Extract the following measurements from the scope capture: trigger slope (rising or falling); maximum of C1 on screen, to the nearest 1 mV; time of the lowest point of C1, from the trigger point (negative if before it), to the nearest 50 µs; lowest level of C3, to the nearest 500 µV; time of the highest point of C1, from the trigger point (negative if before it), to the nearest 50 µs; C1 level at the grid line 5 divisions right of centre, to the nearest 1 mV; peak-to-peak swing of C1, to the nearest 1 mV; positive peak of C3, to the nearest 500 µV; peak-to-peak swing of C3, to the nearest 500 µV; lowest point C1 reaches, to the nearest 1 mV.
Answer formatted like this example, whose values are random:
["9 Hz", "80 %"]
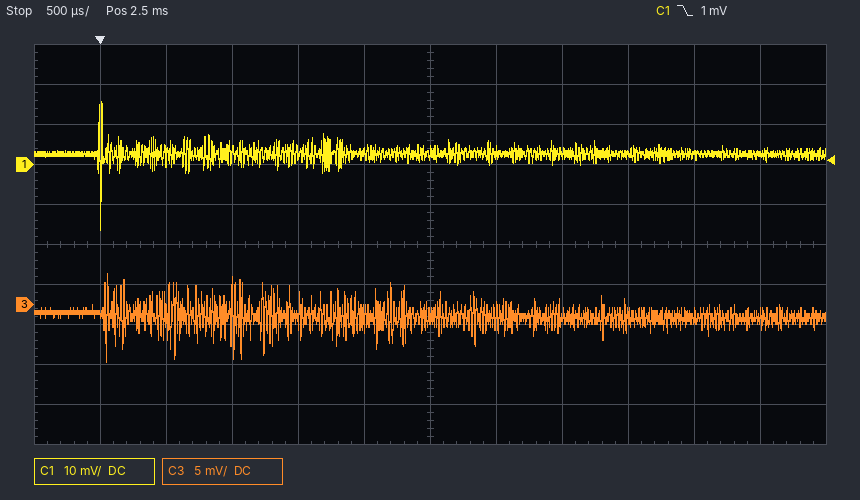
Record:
["falling", "16 mV", "0 µs", "-7.0 mV", "0 µs", "3 mV", "32 mV", "4.0 mV", "11.0 mV", "-16 mV"]
